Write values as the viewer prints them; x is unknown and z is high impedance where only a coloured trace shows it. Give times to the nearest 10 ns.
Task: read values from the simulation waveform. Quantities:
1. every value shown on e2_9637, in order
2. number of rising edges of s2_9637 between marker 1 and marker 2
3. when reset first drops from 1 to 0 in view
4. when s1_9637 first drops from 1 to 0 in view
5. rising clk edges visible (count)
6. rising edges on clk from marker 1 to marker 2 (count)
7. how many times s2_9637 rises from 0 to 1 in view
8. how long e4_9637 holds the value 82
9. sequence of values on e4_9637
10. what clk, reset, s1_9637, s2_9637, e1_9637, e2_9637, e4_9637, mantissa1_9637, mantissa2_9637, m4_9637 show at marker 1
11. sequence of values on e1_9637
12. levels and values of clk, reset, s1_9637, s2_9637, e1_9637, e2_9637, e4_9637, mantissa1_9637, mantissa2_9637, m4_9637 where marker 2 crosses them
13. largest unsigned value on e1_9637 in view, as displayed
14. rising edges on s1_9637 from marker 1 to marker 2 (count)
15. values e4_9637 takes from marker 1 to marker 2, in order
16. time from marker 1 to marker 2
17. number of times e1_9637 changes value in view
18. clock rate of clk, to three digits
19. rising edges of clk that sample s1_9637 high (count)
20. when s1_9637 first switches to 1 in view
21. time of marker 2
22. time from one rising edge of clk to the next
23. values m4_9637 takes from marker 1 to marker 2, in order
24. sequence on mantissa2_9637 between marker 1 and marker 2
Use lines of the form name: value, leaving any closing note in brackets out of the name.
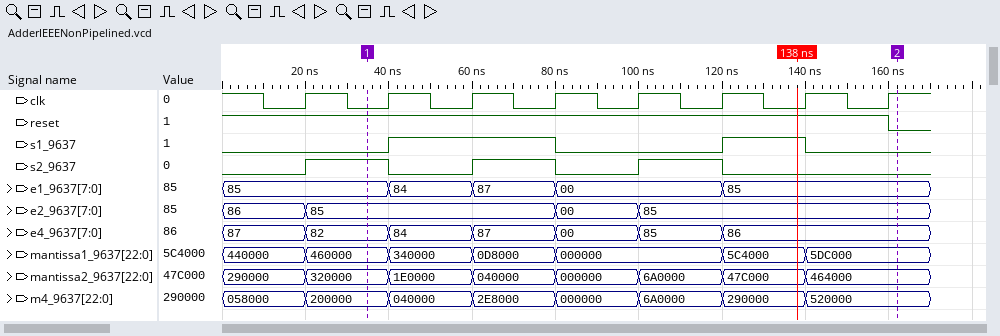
every value shown on e2_9637, in order: 86, 85, 00, 85
number of rising edges of s2_9637 between marker 1 and marker 2: 2
when reset first drops from 1 to 0 in view: 160 ns
when s1_9637 first drops from 1 to 0 in view: 80 ns
rising clk edges visible: 8
rising edges on clk from marker 1 to marker 2: 7
how many times s2_9637 rises from 0 to 1 in view: 3
how long e4_9637 holds the value 82: 20 ns
sequence of values on e4_9637: 87, 82, 84, 87, 00, 85, 86
what clk, reset, s1_9637, s2_9637, e1_9637, e2_9637, e4_9637, mantissa1_9637, mantissa2_9637, m4_9637 show at marker 1: clk=0, reset=1, s1_9637=0, s2_9637=1, e1_9637=85, e2_9637=85, e4_9637=82, mantissa1_9637=460000, mantissa2_9637=320000, m4_9637=200000
sequence of values on e1_9637: 85, 84, 87, 00, 85
levels and values of clk, reset, s1_9637, s2_9637, e1_9637, e2_9637, e4_9637, mantissa1_9637, mantissa2_9637, m4_9637 where marker 2 crosses them: clk=1, reset=0, s1_9637=0, s2_9637=0, e1_9637=85, e2_9637=85, e4_9637=86, mantissa1_9637=5DC000, mantissa2_9637=464000, m4_9637=520000
largest unsigned value on e1_9637 in view, as displayed: 87
rising edges on s1_9637 from marker 1 to marker 2: 2
values e4_9637 takes from marker 1 to marker 2, in order: 82, 84, 87, 00, 85, 86
time from marker 1 to marker 2: 130 ns
number of times e1_9637 changes value in view: 4
clock rate of clk, to three digits: 50.0 MHz
rising edges of clk that sample s1_9637 high: 3
when s1_9637 first switches to 1 in view: 40 ns
time of marker 2: 160 ns
time from one rising edge of clk to the next: 20 ns
values m4_9637 takes from marker 1 to marker 2, in order: 200000, 040000, 2E8000, 000000, 6A0000, 290000, 520000
sequence on mantissa2_9637 between marker 1 and marker 2: 320000, 1E0000, 040000, 000000, 6A0000, 47C000, 464000
